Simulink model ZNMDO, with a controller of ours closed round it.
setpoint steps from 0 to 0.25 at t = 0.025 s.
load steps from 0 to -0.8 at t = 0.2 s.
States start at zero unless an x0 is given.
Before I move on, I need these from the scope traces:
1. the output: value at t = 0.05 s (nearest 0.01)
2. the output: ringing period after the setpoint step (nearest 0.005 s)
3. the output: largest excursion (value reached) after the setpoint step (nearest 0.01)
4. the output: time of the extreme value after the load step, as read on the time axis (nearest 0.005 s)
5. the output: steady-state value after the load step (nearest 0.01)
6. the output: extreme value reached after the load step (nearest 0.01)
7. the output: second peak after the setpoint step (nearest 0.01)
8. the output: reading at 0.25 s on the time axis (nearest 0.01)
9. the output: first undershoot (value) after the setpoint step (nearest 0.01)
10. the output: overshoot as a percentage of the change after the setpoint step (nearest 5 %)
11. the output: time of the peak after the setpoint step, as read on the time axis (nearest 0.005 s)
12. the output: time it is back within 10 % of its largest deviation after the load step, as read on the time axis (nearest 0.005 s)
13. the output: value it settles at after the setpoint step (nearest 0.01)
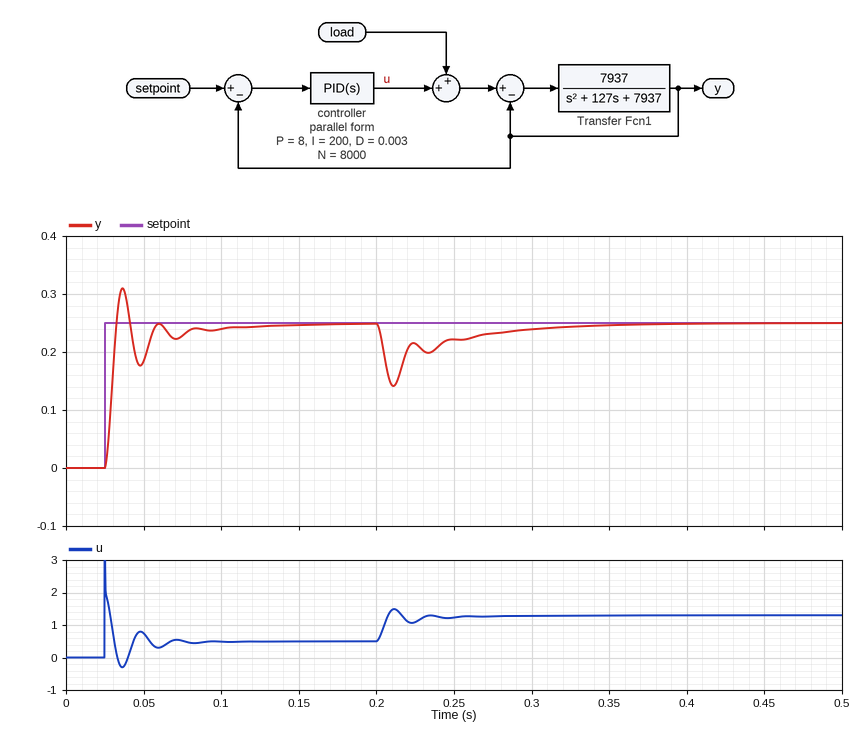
0.18
0.025 s
0.31
0.210 s
0.25
0.14
0.25
0.22
0.18
25 %
0.035 s
0.300 s
0.25
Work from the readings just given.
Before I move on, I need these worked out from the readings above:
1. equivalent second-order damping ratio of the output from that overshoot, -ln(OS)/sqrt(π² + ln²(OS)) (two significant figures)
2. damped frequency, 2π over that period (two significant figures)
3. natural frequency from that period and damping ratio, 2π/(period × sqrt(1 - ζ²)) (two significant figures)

0.40
250 rad/s
270 rad/s
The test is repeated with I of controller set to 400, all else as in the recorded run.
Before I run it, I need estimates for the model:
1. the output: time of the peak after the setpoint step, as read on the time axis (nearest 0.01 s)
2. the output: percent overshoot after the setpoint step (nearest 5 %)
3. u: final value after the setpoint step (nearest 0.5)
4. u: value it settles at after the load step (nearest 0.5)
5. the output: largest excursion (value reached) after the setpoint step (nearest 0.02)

0.04 s
35 %
0.5
1.5
0.34
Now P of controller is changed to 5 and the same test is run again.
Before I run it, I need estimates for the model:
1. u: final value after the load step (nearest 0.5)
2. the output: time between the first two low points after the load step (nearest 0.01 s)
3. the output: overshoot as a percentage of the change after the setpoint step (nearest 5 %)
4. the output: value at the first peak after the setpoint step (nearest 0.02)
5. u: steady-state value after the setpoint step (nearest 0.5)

1.5
0.03 s
15 %
0.28
0.5
